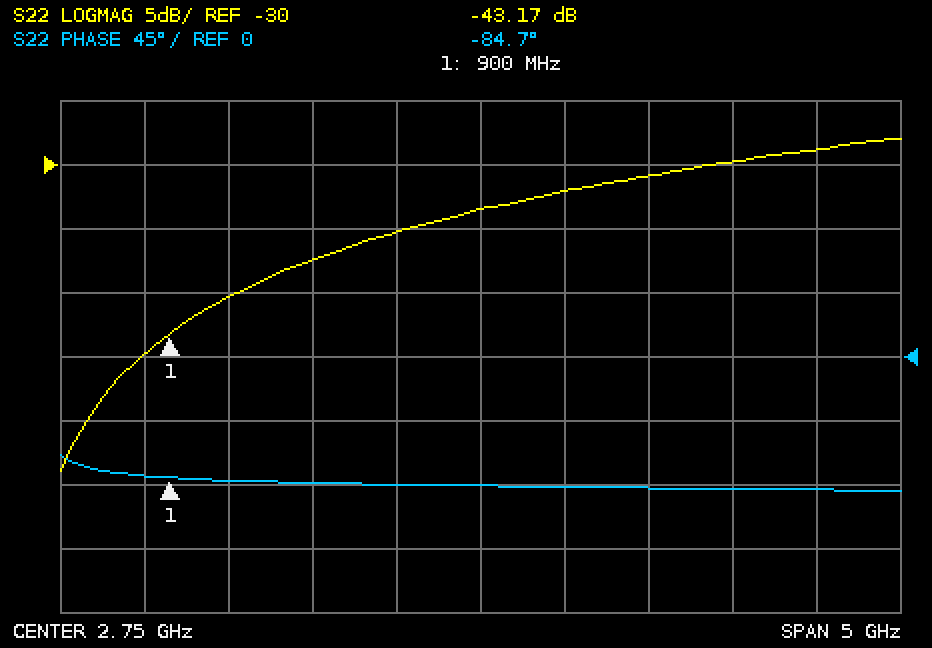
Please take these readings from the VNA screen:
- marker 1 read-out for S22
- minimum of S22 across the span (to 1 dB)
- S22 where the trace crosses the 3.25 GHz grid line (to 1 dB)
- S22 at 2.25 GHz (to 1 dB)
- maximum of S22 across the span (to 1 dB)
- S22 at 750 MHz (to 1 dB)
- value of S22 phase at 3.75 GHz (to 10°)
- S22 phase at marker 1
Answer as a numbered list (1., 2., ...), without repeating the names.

1. -43.17 dB
2. -54 dB
3. -32 dB
4. -35 dB
5. -28 dB
6. -45 dB
7. -90°
8. -84.7°
